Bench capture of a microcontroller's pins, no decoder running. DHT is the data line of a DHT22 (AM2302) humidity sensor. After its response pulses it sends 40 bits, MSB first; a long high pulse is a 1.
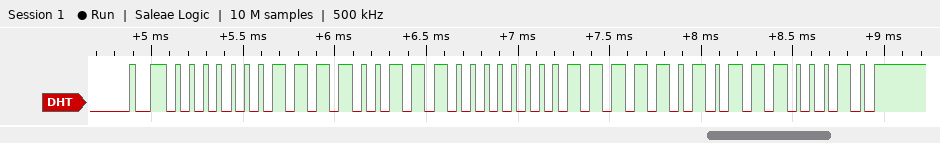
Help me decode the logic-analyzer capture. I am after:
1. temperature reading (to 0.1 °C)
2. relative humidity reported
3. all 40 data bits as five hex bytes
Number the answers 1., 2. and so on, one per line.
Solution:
1. 25.0 °C
2. 48.7 %
3. 01 E7 00 FA E2
